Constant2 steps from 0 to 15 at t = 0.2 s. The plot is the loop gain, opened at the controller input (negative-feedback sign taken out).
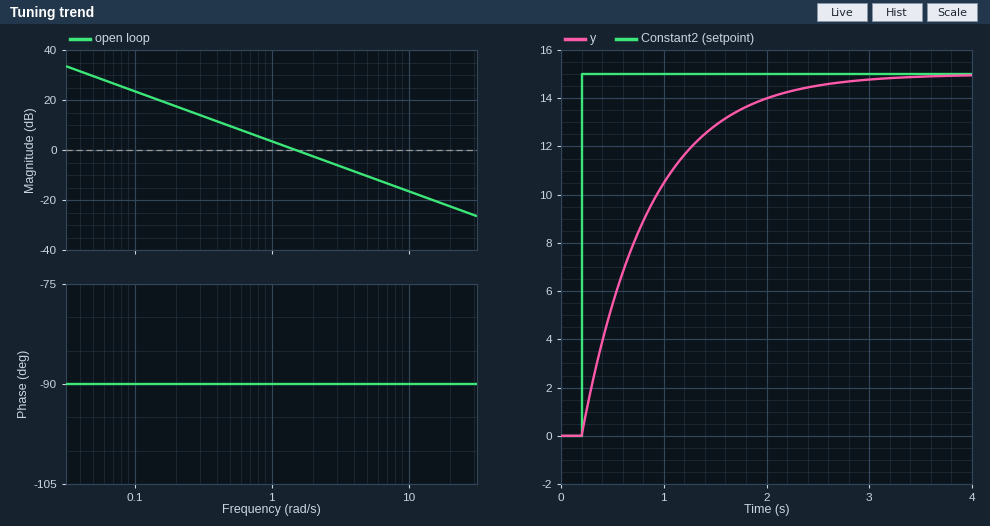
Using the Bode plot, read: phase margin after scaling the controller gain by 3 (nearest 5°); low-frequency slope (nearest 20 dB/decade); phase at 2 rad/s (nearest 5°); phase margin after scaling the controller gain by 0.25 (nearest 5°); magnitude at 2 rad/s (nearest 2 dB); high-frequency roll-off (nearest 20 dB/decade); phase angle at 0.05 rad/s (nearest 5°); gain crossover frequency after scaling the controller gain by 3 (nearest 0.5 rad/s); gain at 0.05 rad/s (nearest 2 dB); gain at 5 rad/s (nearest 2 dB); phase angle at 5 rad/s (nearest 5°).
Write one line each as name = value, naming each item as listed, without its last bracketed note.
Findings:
phase margin after scaling the controller gain by 3 = 90°
low-frequency slope = -20 dB/decade
phase at 2 rad/s = -90°
phase margin after scaling the controller gain by 0.25 = 90°
magnitude at 2 rad/s = -2 dB
high-frequency roll-off = -20 dB/decade
phase angle at 0.05 rad/s = -90°
gain crossover frequency after scaling the controller gain by 3 = 4.5 rad/s
gain at 0.05 rad/s = 30 dB
gain at 5 rad/s = -10 dB
phase angle at 5 rad/s = -90°
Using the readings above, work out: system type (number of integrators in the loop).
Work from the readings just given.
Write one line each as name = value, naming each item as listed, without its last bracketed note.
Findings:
system type = 1
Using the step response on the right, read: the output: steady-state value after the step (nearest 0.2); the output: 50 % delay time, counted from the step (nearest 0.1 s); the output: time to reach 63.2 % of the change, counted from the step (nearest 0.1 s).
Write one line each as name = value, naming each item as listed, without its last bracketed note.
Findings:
the output: steady-state value after the step = 15.0
the output: 50 % delay time, counted from the step = 0.5 s
the output: time to reach 63.2 % of the change, counted from the step = 0.7 s
